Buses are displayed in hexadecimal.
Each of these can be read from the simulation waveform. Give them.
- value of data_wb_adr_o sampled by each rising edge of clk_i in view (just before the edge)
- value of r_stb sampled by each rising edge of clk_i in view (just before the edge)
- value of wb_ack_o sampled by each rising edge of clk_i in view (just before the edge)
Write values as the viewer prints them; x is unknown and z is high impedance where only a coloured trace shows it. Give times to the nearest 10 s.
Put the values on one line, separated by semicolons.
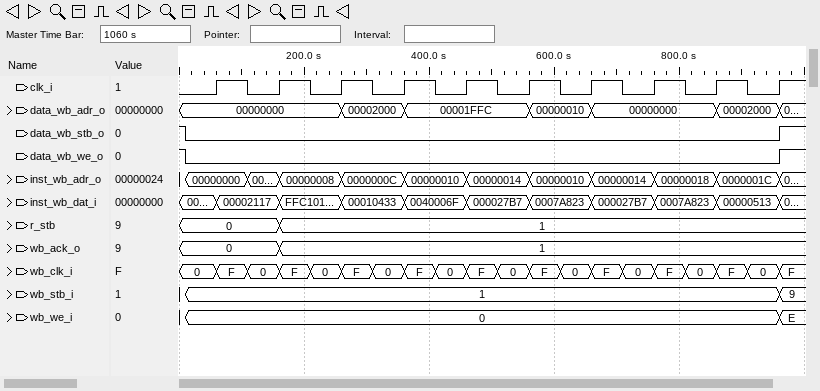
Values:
00000000, 00000000, 00000000, 00002000, 00001FFC, 00001FFC, 00000010, 00000000, 00000000, 00002000; 0, 0, 1, 1, 1, 1, 1, 1, 1, 1; 0, 0, 1, 1, 1, 1, 1, 1, 1, 1
